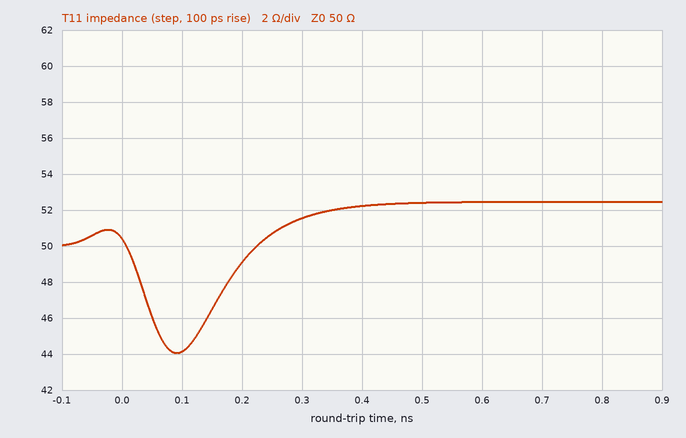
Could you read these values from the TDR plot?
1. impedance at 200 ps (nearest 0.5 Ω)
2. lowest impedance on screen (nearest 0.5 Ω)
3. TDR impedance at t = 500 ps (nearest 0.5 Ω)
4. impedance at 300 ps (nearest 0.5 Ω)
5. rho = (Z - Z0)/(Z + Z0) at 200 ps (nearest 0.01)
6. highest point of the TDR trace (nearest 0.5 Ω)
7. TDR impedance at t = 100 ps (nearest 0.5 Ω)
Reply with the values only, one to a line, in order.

49.0 Ω
44.0 Ω
52.5 Ω
51.5 Ω
-0.01
52.5 Ω
44.0 Ω
